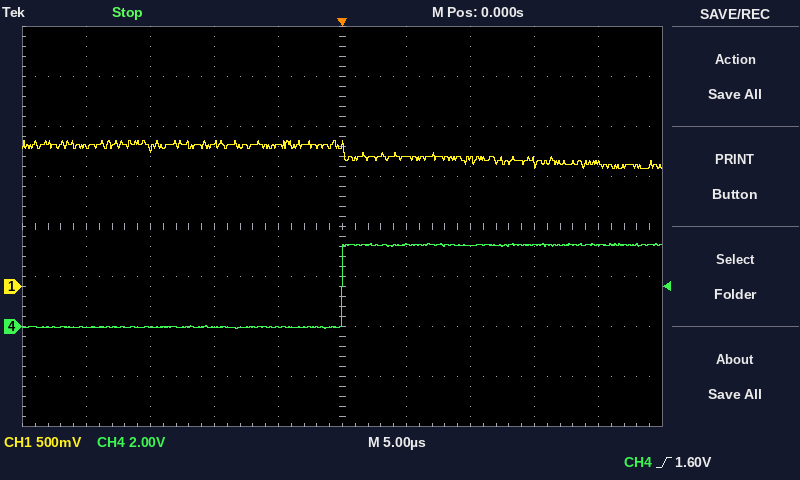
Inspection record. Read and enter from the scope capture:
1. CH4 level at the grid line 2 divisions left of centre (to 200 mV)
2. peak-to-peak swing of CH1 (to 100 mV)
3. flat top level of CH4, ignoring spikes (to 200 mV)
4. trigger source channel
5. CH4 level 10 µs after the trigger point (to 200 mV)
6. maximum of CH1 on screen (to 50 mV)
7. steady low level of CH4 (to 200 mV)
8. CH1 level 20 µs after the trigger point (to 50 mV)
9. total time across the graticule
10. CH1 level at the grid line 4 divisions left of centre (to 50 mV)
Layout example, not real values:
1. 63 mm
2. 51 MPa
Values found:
1. 0.0 V
2. 300 mV
3. 3.2 V
4. CH4
5. 3.2 V
6. 1.45 V
7. 0.0 V
8. 1.25 V
9. 50 µs
10. 1.40 V
